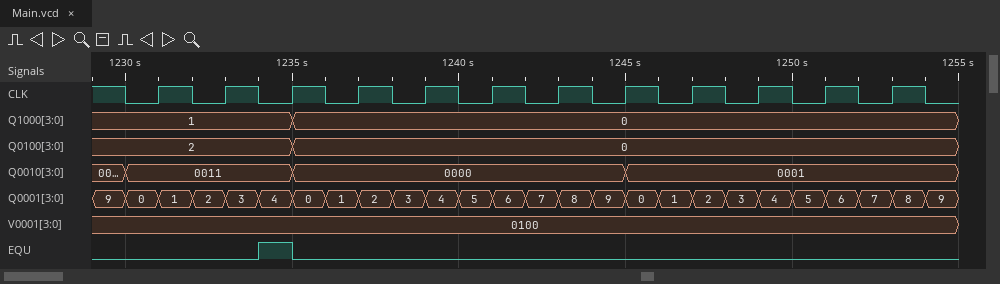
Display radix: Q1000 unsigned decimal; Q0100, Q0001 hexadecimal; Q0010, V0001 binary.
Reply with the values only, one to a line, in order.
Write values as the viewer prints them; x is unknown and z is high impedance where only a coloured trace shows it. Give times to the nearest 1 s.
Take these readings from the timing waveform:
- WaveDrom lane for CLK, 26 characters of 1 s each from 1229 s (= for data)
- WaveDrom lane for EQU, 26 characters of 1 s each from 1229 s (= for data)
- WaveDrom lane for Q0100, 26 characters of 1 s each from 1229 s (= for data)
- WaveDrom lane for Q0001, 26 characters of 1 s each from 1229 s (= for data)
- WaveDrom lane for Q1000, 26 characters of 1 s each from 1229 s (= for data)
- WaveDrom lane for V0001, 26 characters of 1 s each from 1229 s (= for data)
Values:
{name: 'CLK', wave: '10101010101010101010101010'}
{name: 'EQU', wave: '0....10...................'}
{name: 'Q0100', wave: '=.....=...................', data: '2 0'}
{name: 'Q0001', wave: '==========================', data: '9 0 1 2 3 4 0 1 2 3 4 5 6 7 8 9 0 1 2 3 4 5 6 7 8 9'}
{name: 'Q1000', wave: '=.....=...................', data: '1 0'}
{name: 'V0001', wave: '=.........................', data: '0100'}
